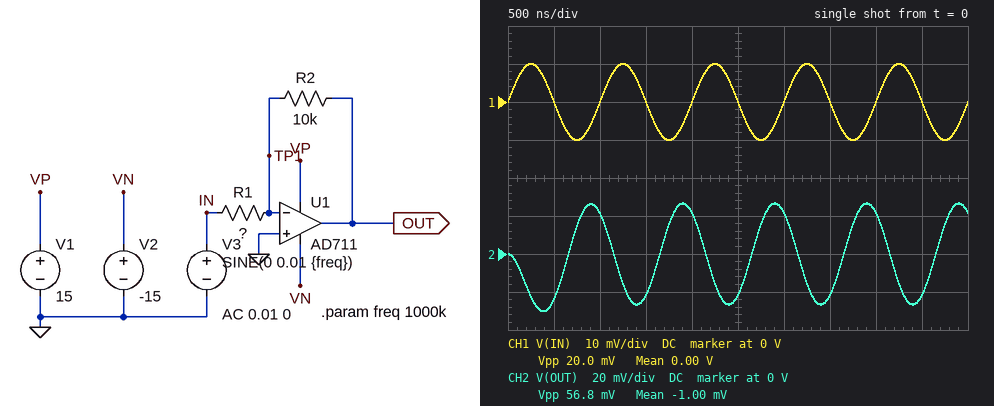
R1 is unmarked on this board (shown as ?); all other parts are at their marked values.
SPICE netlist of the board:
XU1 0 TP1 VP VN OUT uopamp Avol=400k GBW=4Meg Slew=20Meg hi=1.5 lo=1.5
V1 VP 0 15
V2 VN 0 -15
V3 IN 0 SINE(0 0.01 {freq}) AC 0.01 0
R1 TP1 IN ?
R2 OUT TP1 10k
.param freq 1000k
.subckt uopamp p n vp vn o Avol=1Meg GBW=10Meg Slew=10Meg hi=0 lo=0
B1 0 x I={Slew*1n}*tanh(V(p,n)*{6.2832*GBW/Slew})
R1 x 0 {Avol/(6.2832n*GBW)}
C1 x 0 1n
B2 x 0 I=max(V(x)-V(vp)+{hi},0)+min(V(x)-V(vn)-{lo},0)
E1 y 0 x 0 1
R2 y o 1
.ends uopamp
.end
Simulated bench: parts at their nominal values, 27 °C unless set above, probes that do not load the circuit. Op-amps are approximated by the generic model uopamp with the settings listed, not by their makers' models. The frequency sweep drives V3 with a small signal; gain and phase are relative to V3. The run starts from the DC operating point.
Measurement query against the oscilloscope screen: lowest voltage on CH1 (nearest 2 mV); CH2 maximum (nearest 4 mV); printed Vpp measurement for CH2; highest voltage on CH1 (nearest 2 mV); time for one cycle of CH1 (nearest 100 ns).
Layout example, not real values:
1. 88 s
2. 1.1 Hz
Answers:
1. -10 mV
2. 28 mV
3. 56.8 mV
4. 10 mV
5. 1.0 µs
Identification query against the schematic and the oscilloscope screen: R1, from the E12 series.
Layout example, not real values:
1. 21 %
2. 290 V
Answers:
1. 2.2 kΩ
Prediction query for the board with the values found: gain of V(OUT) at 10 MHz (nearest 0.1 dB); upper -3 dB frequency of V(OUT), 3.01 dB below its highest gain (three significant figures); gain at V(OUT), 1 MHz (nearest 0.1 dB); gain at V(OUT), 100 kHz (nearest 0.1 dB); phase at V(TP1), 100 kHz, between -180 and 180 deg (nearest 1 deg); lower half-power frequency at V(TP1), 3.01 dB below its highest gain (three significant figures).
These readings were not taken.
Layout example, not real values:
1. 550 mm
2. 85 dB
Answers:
1. -9.7 dB
2. 721 kHz
3. 8.5 dB
4. 13.1 dB
5. 82 deg
6. 721 kHz
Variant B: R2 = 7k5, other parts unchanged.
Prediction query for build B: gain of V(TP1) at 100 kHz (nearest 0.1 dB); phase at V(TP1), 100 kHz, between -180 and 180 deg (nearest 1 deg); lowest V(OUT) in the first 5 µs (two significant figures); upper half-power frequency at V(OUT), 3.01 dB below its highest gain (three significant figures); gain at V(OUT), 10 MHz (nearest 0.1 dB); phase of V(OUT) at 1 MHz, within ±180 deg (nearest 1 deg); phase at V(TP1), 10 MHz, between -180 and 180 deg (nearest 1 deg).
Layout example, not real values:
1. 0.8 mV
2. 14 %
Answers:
1. -21.4 dB
2. 84 deg
3. -25 mV
4. 907 kHz
5. -10.2 dB
6. 132 deg
7. 5 deg
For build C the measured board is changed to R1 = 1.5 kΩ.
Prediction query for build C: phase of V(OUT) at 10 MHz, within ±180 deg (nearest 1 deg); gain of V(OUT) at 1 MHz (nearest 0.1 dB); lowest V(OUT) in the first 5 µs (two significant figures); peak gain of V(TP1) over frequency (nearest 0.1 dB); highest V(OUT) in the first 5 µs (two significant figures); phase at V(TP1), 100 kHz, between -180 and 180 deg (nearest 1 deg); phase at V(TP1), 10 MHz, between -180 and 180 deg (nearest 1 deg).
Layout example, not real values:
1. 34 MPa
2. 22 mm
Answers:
1. 93 deg
2. 9.8 dB
3. -38 mV
4. -1.2 dB
5. 31 mV
6. 79 deg
7. 3 deg
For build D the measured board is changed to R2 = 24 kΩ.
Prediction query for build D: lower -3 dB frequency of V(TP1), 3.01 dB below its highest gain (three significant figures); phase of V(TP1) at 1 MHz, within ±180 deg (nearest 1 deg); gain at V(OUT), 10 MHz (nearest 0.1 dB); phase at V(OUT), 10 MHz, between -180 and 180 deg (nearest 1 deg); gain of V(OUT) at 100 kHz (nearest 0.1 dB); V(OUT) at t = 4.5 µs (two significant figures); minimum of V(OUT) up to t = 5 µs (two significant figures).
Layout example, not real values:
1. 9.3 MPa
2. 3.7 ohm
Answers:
1. 336 kHz
2. 19 deg
3. -8.7 dB
4. 92 deg
5. 20.4 dB
6. -33 mV
7. -48 mV
